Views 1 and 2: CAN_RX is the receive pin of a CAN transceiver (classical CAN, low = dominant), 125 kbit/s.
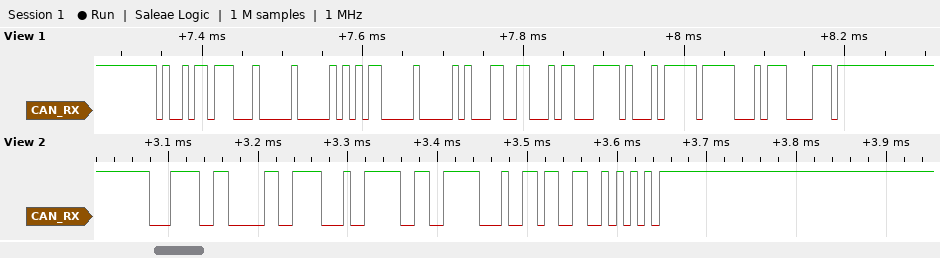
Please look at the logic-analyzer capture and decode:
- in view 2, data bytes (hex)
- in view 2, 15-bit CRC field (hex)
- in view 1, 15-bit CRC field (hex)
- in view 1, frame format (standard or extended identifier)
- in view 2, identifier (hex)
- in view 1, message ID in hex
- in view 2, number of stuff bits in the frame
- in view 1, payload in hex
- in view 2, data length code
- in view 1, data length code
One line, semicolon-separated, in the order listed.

F1 3E CF 93; 0x332A; 0x65C3; standard; 0x1E6; 0x4B7; 3; 00 AC 00 46 62 C7 A2 FF; 4; 8
